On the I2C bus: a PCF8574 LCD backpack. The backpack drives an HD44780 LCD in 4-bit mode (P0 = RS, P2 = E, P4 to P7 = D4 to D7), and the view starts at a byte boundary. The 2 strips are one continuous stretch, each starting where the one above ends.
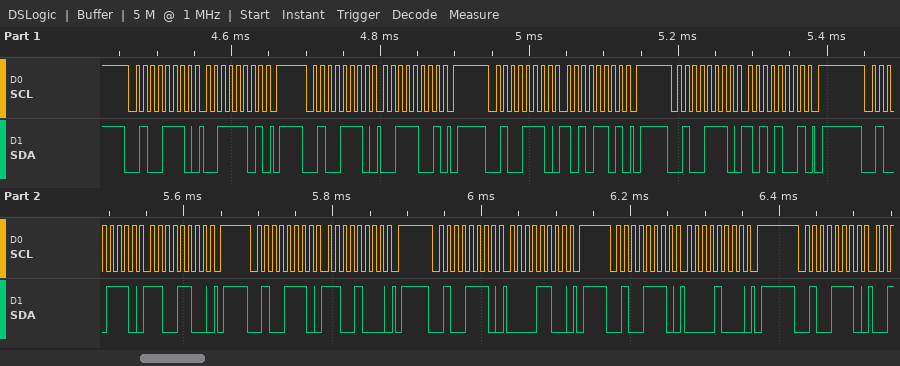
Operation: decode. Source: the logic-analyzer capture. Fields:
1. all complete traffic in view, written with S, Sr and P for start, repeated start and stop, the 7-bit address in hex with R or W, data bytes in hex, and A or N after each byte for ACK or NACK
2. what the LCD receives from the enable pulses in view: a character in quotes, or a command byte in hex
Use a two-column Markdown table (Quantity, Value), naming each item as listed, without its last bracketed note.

| Quantity | Value |
|---|---|
| all complete traffic in view, written with S, Sr and P for start, repeated start and stop, the 7-bit address in hex with R or W, data bytes in hex, and A or N after each byte for ACK or NACK | S 27W A 3D A P S 27W A 39 A P S 27W A AD A P S 27W A A9 A P S 27W A CC A P S 27W A C8 A P S 27W A 0C A P S 27W A 08 A P S 27W A |
| what the LCD receives from the enable pulses in view: a character in quotes, or a command byte in hex | ':' 0xC0 |
